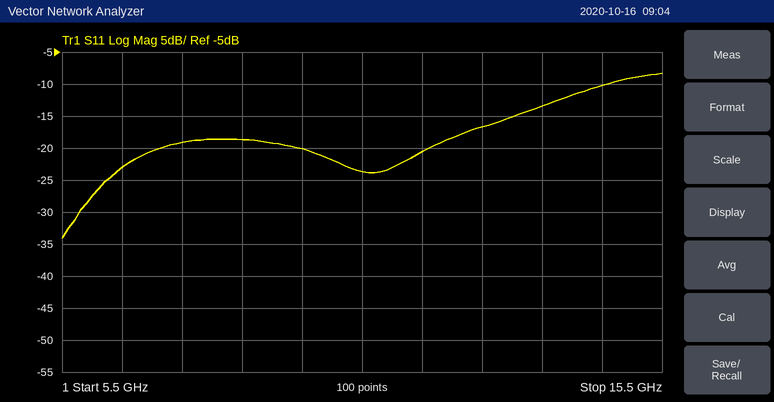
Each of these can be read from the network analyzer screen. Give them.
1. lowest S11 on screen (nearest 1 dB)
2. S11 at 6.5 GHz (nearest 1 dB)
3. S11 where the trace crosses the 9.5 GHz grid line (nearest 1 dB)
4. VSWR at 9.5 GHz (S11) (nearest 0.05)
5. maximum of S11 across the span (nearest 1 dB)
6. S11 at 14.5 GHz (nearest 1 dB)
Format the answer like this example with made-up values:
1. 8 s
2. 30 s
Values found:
1. -34 dB
2. -23 dB
3. -20 dB
4. 1.20
5. -8 dB
6. -10 dB
